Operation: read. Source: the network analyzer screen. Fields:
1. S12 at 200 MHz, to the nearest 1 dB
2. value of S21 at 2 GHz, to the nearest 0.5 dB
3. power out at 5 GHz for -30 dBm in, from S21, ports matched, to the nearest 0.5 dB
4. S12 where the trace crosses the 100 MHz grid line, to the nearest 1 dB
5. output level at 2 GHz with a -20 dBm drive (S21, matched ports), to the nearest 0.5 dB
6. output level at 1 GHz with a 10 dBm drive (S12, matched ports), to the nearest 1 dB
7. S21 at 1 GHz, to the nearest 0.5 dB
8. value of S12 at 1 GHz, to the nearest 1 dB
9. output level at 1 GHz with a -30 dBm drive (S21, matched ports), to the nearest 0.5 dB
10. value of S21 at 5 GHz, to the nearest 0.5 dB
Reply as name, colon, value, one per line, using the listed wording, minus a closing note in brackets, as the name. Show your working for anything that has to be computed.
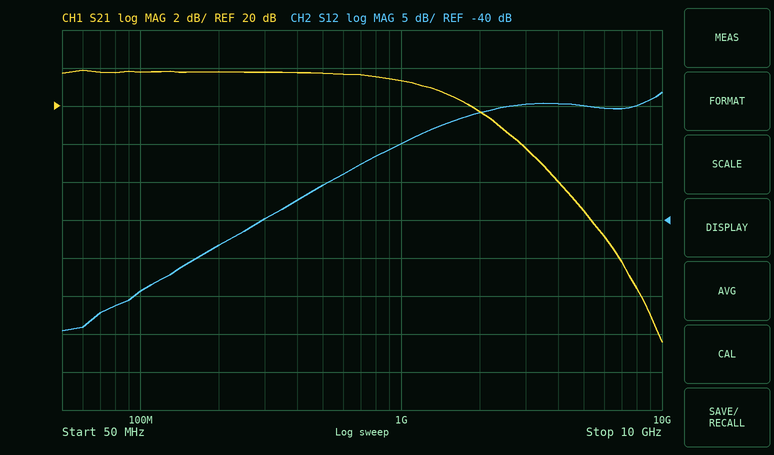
S12 at 200 MHz, to the nearest 1 dB: -43 dB
value of S21 at 2 GHz, to the nearest 0.5 dB: 19.5 dB
power out at 5 GHz for -30 dBm in, from S21, ports matched, to the nearest 0.5 dB: -30 dBm + (14.5 dB) = -15.5 dBm
S12 where the trace crosses the 100 MHz grid line, to the nearest 1 dB: -49 dB
output level at 2 GHz with a -20 dBm drive (S21, matched ports), to the nearest 0.5 dB: -20 dBm + (19.5 dB) = -0.5 dBm
output level at 1 GHz with a 10 dBm drive (S12, matched ports), to the nearest 1 dB: 10 dBm + (-30 dB) = -20 dBm
S21 at 1 GHz, to the nearest 0.5 dB: 21.5 dB
value of S12 at 1 GHz, to the nearest 1 dB: -30 dB
output level at 1 GHz with a -30 dBm drive (S21, matched ports), to the nearest 0.5 dB: -30 dBm + (21.5 dB) = -8.5 dBm
value of S21 at 5 GHz, to the nearest 0.5 dB: 14.5 dB
